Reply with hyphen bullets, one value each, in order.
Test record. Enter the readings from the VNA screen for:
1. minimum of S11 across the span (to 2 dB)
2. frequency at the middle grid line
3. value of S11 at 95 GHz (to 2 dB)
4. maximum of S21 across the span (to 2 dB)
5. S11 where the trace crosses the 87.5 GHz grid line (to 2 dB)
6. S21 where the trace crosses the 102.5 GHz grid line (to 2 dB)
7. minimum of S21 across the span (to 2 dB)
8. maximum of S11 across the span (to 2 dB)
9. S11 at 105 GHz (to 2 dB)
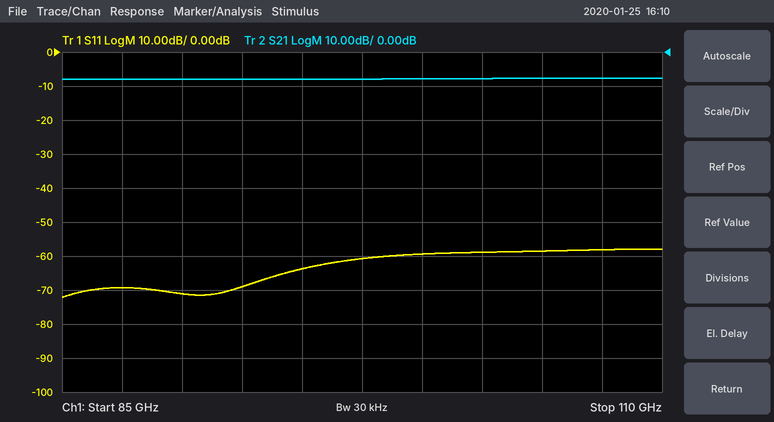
- -72 dB
- 97.5 GHz
- -64 dB
- -8 dB
- -70 dB
- -8 dB
- -8 dB
- -58 dB
- -58 dB
